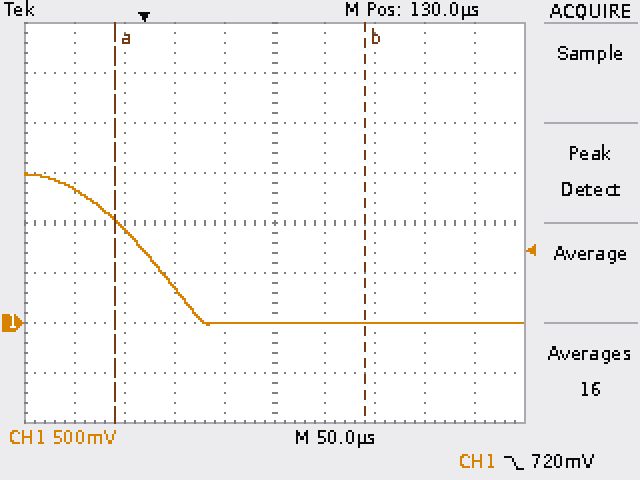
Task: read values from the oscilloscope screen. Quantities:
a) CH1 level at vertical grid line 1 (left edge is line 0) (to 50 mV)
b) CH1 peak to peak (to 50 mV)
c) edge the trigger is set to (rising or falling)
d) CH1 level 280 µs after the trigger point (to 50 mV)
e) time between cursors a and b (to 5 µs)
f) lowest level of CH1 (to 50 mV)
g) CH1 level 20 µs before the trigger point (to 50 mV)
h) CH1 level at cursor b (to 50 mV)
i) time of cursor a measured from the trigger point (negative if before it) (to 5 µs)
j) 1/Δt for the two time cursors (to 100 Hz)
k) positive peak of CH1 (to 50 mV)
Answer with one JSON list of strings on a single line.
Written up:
["1.35 V", "1.50 V", "falling", "0 mV", "250 µs", "0 mV", "950 mV", "0 mV", "-30 µs", "4.0 kHz", "1.50 V"]
